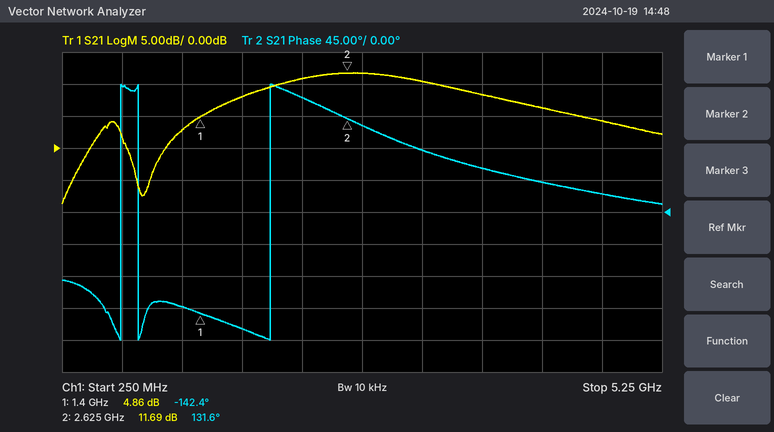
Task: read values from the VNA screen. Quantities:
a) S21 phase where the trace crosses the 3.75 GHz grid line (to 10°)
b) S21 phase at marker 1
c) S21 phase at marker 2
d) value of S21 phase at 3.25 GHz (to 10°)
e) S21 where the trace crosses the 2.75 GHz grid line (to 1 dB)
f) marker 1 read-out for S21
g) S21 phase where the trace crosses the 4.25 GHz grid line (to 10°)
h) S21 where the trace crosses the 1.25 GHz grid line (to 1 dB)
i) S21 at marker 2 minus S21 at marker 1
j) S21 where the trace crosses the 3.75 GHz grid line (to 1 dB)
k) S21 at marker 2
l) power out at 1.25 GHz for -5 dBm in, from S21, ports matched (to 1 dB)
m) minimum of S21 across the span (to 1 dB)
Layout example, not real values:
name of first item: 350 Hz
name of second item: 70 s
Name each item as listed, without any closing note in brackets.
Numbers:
S21 phase where the trace crosses the 3.75 GHz grid line: 60°
S21 phase at marker 1: -142.4°
S21 phase at marker 2: 131.6°
value of S21 phase at 3.25 GHz: 90°
S21 where the trace crosses the 2.75 GHz grid line: 12 dB
marker 1 read-out for S21: 4.86 dB
S21 phase where the trace crosses the 4.25 GHz grid line: 40°
S21 where the trace crosses the 1.25 GHz grid line: 3 dB
S21 at marker 2 minus S21 at marker 1: 6.83 dB
S21 where the trace crosses the 3.75 GHz grid line: 8 dB
S21 at marker 2: 11.69 dB
power out at 1.25 GHz for -5 dBm in, from S21, ports matched: -2 dBm
minimum of S21 across the span: -9 dB
